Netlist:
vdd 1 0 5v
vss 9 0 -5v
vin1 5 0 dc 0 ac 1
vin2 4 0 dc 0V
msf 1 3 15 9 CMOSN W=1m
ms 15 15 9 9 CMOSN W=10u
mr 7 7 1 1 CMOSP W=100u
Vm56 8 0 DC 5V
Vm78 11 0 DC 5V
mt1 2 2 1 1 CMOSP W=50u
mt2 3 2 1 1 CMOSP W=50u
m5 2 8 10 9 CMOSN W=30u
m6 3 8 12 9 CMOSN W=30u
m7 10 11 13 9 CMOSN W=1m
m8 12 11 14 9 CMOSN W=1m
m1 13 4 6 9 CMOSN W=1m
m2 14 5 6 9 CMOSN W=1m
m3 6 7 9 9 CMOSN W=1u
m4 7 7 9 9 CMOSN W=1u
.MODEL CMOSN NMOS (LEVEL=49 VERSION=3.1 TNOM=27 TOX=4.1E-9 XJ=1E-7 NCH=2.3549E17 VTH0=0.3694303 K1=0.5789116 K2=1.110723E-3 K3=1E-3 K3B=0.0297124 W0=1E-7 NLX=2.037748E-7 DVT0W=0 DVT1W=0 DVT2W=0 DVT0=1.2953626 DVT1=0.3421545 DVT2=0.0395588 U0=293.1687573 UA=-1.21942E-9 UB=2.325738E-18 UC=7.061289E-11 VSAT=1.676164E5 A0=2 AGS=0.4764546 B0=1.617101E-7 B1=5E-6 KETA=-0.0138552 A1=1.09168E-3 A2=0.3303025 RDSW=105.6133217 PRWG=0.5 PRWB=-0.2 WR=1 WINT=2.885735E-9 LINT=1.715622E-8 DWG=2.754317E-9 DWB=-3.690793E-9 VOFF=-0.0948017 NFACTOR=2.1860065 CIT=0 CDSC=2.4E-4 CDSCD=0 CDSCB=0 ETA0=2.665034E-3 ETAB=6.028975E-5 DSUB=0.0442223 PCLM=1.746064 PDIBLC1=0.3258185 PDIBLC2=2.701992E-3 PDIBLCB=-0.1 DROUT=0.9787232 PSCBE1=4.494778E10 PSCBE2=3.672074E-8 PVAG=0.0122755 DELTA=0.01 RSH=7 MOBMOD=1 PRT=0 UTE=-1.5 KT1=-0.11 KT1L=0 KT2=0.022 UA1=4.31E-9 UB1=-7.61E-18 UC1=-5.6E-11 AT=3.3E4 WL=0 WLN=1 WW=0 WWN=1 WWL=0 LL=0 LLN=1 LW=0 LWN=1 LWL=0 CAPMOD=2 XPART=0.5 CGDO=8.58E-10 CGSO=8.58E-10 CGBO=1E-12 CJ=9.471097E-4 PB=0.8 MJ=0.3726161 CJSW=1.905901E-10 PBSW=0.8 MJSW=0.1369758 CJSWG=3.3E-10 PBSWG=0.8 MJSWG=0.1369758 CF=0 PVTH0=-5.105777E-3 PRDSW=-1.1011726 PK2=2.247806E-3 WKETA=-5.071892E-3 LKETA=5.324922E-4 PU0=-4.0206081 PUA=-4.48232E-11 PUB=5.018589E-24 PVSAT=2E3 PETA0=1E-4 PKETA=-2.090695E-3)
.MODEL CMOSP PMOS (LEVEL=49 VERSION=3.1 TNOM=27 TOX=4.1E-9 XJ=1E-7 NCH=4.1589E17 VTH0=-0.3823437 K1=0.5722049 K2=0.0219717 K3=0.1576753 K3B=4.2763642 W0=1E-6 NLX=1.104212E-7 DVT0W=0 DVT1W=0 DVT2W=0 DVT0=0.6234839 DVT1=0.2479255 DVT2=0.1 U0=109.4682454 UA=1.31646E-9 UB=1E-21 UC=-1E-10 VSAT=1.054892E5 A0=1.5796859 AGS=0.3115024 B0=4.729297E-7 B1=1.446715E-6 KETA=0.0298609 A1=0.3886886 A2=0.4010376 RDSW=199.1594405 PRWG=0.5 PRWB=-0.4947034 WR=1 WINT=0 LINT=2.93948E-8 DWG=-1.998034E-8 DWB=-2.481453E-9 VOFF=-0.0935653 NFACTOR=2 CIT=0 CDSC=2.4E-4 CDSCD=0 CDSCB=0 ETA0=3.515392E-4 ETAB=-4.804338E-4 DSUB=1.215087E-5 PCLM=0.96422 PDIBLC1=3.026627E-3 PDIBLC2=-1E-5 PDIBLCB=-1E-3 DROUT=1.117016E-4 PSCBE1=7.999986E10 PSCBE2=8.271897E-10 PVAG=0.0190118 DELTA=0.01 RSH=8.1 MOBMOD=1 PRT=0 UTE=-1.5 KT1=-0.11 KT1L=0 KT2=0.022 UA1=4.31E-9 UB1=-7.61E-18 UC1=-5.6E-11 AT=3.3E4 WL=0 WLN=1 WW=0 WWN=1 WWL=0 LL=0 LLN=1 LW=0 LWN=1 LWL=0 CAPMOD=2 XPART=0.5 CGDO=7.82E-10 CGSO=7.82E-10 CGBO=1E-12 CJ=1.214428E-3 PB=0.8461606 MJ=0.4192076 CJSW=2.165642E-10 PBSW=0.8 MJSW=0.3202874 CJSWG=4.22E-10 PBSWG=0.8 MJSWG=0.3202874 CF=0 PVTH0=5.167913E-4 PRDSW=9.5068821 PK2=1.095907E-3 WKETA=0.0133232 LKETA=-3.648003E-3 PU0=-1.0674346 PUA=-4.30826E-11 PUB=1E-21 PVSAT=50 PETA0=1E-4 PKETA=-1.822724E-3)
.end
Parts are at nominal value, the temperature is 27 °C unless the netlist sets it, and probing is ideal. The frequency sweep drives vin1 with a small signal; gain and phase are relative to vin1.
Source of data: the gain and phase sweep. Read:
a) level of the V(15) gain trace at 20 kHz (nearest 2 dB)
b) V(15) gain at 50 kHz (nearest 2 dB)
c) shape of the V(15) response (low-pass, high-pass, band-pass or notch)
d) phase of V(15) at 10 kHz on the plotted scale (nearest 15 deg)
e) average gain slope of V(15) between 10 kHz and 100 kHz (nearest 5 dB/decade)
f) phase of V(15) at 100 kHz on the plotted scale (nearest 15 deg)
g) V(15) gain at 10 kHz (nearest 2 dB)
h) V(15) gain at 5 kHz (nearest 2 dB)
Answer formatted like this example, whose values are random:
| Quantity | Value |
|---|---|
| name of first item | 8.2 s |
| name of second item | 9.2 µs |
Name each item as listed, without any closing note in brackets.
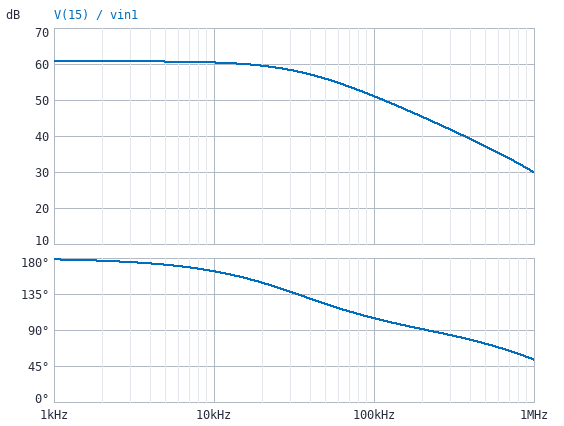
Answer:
| Quantity | Value |
|---|---|
| level of the V(15) gain trace at 20 kHz | 60 dB |
| V(15) gain at 50 kHz | 56 dB |
| shape of the V(15) response | low-pass |
| phase of V(15) at 10 kHz on the plotted scale | 165 deg |
| average gain slope of V(15) between 10 kHz and 100 kHz | -10 dB/decade |
| phase of V(15) at 100 kHz on the plotted scale | 105 deg |
| V(15) gain at 10 kHz | 60 dB |
| V(15) gain at 5 kHz | 60 dB |
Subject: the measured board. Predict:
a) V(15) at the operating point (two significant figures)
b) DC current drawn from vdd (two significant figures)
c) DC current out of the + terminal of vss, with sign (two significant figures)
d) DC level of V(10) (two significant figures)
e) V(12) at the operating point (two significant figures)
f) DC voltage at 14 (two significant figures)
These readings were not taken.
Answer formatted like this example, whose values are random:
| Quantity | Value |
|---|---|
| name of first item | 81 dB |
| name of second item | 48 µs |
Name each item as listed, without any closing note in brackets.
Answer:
| Quantity | Value |
|---|---|
| V(15) at the operating point | 2.2 V |
| DC current drawn from vdd | 3.8 mA |
| DC current out of the + terminal of vss, with sign | -3.8 mA |
| DC level of V(10) | 3.1 V |
| V(12) at the operating point | 3.1 V |
| DC voltage at 14 | 3.1 V |
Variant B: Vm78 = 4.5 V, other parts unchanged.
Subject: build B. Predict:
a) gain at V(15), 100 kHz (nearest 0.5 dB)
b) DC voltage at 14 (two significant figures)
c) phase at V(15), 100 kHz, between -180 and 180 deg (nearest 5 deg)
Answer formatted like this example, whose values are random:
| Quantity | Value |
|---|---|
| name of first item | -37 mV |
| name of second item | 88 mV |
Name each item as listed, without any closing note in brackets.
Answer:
| Quantity | Value |
|---|---|
| gain at V(15), 100 kHz | 51.5 dB |
| DC voltage at 14 | 2.9 V |
| phase at V(15), 100 kHz, between -180 and 180 deg | 110 deg |
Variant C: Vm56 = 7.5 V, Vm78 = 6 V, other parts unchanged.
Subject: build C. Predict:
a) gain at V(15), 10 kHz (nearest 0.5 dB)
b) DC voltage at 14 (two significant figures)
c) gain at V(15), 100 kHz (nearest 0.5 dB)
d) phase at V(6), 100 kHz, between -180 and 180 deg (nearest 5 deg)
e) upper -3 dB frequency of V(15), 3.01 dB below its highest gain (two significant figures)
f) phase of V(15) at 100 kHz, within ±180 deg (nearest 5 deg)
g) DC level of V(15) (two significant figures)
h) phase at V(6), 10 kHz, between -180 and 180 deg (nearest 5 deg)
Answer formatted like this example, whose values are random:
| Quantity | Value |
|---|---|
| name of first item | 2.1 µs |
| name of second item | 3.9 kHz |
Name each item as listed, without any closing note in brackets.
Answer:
| Quantity | Value |
|---|---|
| gain at V(15), 10 kHz | 48.5 dB |
| DC voltage at 14 | 4.0 V |
| gain at V(15), 100 kHz | 32.5 dB |
| phase at V(6), 100 kHz, between -180 and 180 deg | 5 deg |
| upper -3 dB frequency of V(15), 3.01 dB below its highest gain | 12 kHz |
| phase of V(15) at 100 kHz, within ±180 deg | 95 deg |
| DC level of V(15) | 2.2 V |
| phase at V(6), 10 kHz, between -180 and 180 deg | 30 deg |
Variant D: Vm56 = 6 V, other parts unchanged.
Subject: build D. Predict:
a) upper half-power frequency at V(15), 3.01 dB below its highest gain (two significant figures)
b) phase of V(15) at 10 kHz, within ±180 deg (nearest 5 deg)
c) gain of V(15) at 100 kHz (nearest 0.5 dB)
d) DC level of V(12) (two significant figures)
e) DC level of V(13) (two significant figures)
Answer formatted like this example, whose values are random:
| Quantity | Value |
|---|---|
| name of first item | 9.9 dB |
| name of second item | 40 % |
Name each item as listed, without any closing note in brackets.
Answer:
| Quantity | Value |
|---|---|
| upper half-power frequency at V(15), 3.01 dB below its highest gain | 28 kHz |
| phase of V(15) at 10 kHz, within ±180 deg | 160 deg |
| gain of V(15) at 100 kHz | 49.5 dB |
| DC level of V(12) | 3.9 V |
| DC level of V(13) | 3.4 V |
